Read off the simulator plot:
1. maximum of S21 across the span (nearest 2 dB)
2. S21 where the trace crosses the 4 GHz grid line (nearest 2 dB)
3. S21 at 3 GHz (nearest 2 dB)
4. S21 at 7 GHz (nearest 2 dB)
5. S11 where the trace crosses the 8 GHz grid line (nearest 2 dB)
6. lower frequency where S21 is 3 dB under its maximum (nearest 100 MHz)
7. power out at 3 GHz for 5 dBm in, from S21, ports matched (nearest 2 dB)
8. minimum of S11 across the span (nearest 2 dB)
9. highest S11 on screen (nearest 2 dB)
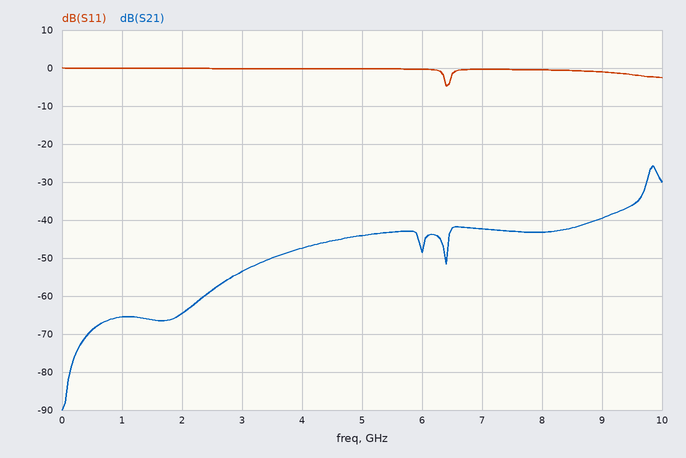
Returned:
-26 dB
-48 dB
-54 dB
-42 dB
0 dB
9.8 GHz
-48 dBm
-4 dB
0 dB
